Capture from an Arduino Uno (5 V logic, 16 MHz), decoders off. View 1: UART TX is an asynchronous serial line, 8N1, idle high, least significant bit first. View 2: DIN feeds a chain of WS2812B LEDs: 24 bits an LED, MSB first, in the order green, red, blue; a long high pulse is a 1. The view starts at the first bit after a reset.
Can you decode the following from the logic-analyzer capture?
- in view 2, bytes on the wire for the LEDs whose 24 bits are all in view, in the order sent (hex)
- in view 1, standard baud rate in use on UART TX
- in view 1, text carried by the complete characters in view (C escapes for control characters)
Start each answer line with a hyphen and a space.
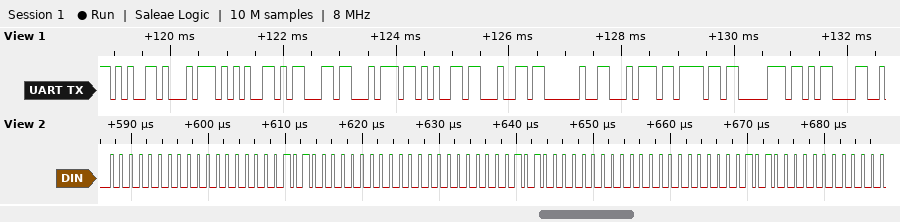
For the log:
- 00 00 28 00 00 28 00 00 28
- 9600 baud
- "etected top\r"
